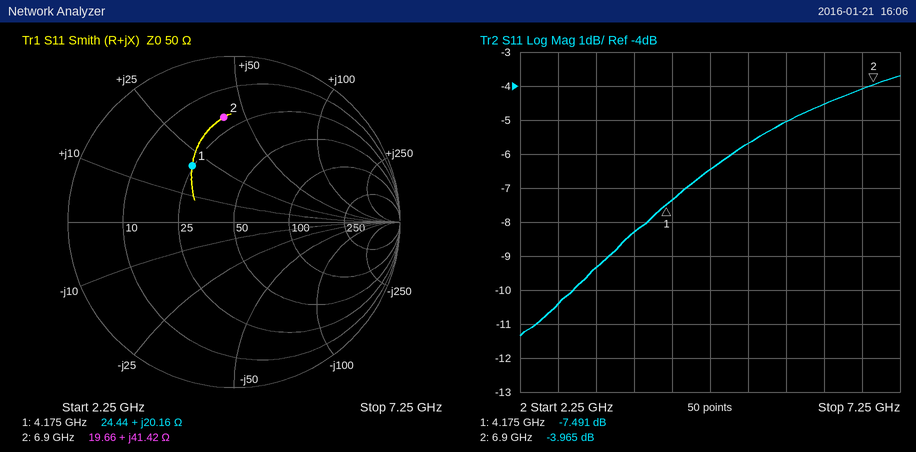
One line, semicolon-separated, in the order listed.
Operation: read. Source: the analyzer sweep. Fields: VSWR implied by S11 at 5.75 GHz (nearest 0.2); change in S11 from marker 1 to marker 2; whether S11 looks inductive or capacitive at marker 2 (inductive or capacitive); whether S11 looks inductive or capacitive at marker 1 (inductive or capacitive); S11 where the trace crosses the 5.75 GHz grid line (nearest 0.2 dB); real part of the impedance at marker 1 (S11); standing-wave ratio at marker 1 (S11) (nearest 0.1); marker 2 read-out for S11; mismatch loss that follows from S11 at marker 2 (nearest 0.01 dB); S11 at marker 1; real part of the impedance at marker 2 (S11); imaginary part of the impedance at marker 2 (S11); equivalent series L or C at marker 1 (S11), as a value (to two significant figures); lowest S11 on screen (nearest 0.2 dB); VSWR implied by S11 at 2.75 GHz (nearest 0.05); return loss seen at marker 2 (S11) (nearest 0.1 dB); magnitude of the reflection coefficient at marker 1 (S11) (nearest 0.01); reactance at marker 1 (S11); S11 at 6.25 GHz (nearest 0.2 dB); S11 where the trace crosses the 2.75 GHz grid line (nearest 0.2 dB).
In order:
3.6; 3.526 dB; inductive; inductive; -5.0 dB; 24.44 Ω; 2.5; -3.965 dB; 2.23 dB; -7.491 dB; 19.66 Ω; +41.42 Ω; 770 pH; -11.4 dB; 1.85; 4.0 dB; 0.42; +20.16 Ω; -4.6 dB; -10.4 dB
